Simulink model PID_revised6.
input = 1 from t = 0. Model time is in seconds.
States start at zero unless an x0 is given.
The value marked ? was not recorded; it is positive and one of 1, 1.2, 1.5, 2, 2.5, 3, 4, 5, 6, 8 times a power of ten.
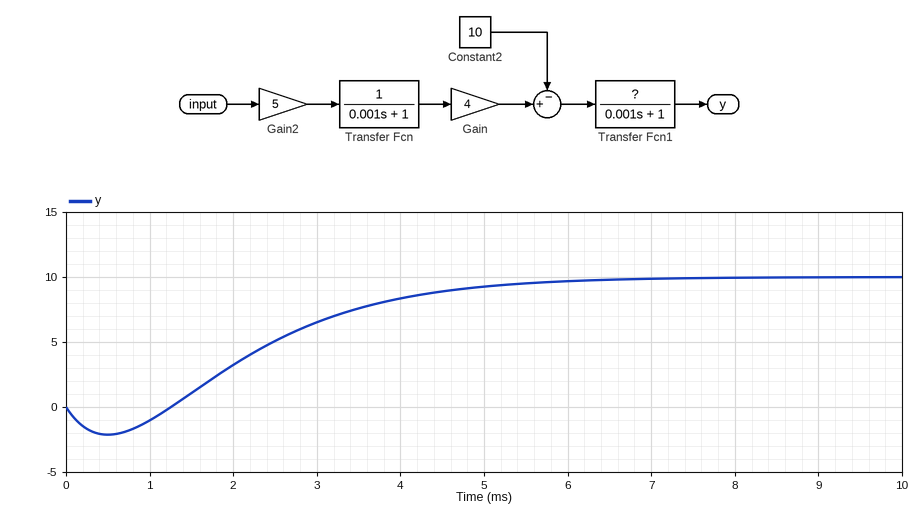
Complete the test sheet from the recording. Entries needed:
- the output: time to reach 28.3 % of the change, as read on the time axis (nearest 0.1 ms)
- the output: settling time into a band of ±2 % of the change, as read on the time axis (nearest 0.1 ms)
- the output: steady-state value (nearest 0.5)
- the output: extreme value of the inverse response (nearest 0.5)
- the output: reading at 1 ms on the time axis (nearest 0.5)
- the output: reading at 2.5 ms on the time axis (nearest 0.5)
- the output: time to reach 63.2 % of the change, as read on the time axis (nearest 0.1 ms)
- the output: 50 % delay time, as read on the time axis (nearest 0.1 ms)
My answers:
1.9 ms
6.6 ms
10.0
-2.0
-1.0
5.0
2.9 ms
2.5 ms
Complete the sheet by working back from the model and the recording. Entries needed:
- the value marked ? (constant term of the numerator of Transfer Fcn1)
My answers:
1
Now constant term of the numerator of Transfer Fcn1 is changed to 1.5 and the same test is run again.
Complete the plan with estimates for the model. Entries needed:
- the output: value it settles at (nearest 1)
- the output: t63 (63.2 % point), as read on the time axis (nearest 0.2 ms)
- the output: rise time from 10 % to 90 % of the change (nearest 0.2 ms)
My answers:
15
3.0 ms
3.2 ms
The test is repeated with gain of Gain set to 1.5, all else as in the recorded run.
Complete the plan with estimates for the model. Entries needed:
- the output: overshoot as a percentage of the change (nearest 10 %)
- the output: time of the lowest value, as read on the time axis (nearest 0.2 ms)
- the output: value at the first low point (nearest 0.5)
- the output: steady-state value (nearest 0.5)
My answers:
80 %
1.4 ms
-4.5
-2.5
